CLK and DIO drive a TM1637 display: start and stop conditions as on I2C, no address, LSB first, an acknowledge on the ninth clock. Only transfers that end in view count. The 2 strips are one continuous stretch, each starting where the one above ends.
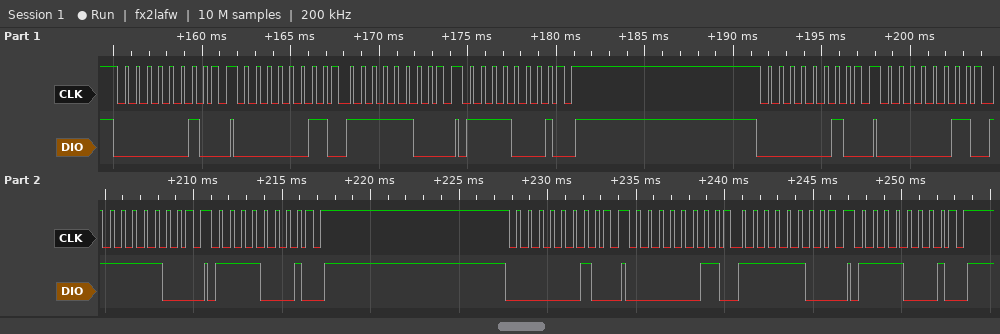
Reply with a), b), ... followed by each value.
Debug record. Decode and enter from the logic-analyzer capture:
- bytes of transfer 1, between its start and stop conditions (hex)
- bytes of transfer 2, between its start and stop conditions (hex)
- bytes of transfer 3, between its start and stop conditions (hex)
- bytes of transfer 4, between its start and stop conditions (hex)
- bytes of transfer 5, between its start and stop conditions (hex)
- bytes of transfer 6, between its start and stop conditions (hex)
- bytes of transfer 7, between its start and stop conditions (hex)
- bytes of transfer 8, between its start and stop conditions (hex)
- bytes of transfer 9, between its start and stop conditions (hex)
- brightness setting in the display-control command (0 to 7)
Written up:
a) 40
b) C0 3F
c) 8F
d) 40
e) C0 3F
f) 8F
g) 40
h) C0 3F
i) 8F
j) 7
